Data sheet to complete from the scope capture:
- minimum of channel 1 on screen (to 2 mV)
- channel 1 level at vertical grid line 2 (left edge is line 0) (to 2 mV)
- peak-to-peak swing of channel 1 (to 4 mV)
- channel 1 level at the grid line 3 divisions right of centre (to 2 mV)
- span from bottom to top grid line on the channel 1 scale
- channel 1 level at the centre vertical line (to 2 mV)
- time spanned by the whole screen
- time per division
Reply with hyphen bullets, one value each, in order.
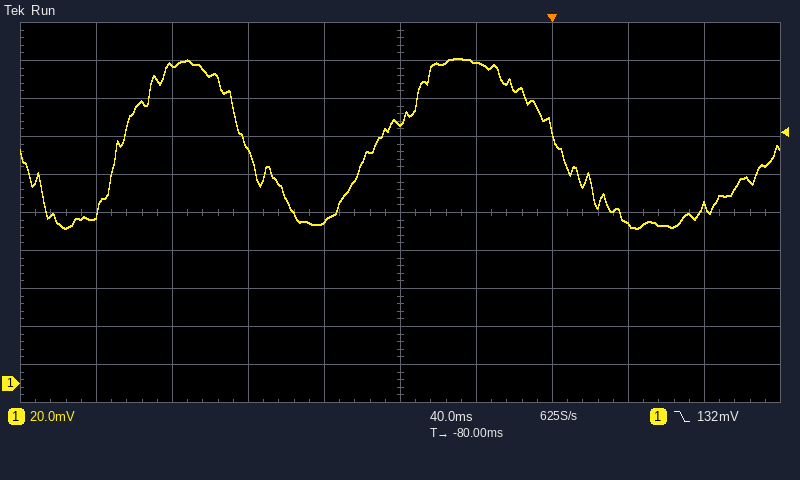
- 82 mV
- 168 mV
- 88 mV
- 84 mV
- 200 mV
- 138 mV
- 400 ms
- 40 ms
